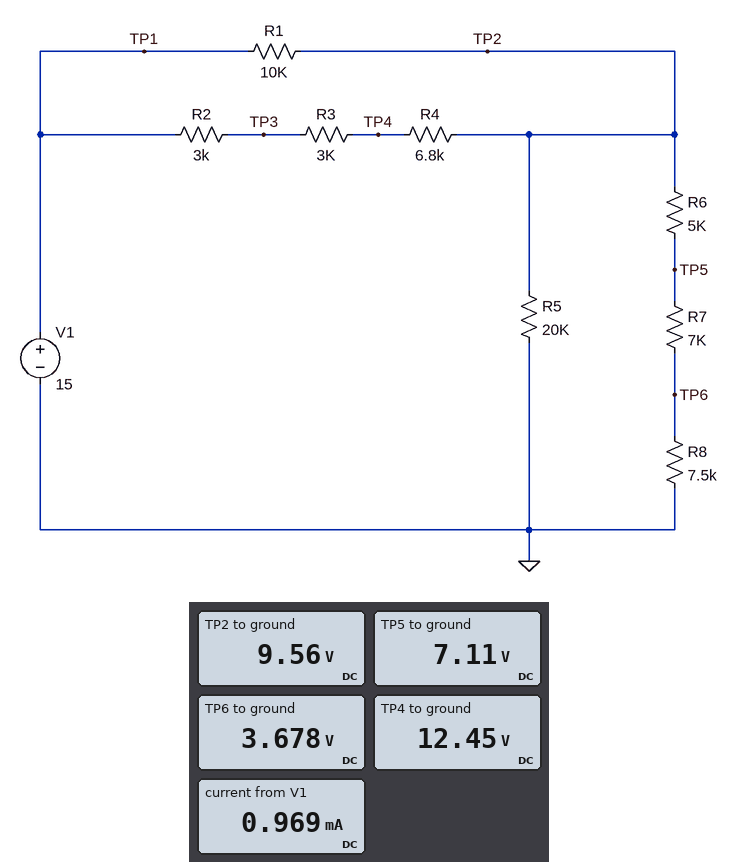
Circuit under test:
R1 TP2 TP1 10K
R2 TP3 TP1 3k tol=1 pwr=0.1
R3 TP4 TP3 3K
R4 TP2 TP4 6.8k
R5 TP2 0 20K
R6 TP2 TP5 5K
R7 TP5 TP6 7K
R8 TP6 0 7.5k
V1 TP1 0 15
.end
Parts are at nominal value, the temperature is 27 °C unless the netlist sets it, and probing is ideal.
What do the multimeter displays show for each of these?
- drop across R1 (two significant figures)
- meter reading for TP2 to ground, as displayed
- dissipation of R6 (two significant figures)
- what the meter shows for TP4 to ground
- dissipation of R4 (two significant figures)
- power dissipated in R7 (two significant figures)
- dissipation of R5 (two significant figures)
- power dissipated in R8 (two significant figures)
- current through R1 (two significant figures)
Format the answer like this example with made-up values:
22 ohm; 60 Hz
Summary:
5.4 V; 9.56 V; 1.2 mW; 12.45 V; 1.2 mW; 1.7 mW; 4.6 mW; 1.8 mW; 540 µA
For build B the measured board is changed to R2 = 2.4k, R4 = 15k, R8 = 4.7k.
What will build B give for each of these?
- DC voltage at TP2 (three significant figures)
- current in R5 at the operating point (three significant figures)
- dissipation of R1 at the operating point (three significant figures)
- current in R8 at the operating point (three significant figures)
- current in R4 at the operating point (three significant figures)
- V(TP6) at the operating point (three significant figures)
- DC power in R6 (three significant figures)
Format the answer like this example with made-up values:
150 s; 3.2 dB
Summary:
8.63 V; 432 µA; 4.05 mW; 517 µA; 312 µA; 2.43 V; 1.34 mW
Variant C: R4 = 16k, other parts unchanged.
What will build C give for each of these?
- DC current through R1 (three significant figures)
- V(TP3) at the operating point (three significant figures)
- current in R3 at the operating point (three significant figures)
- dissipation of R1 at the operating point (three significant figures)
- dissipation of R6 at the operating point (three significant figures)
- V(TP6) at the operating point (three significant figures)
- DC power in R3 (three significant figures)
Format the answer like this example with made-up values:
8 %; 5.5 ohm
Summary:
616 µA; 14.2 V; 280 µA; 3.79 mW; 1.03 mW; 3.40 V; 235 µW
